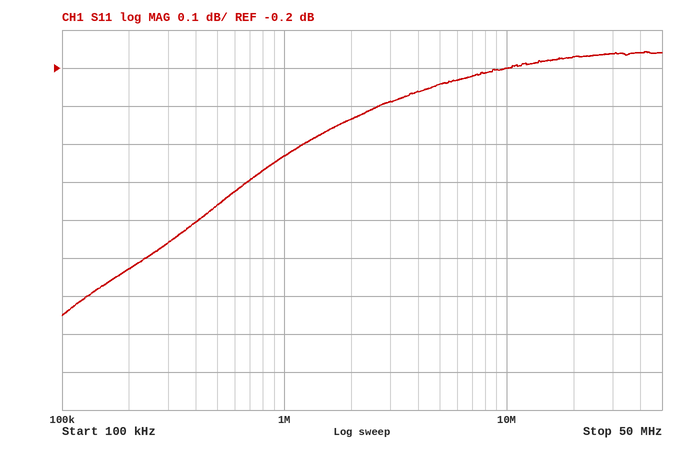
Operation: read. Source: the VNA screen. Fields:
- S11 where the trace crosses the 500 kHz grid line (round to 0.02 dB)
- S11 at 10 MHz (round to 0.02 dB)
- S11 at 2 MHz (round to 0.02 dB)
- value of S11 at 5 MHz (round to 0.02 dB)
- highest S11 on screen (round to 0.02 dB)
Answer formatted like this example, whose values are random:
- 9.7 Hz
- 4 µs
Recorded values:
- -0.56 dB
- -0.20 dB
- -0.34 dB
- -0.24 dB
- -0.16 dB
